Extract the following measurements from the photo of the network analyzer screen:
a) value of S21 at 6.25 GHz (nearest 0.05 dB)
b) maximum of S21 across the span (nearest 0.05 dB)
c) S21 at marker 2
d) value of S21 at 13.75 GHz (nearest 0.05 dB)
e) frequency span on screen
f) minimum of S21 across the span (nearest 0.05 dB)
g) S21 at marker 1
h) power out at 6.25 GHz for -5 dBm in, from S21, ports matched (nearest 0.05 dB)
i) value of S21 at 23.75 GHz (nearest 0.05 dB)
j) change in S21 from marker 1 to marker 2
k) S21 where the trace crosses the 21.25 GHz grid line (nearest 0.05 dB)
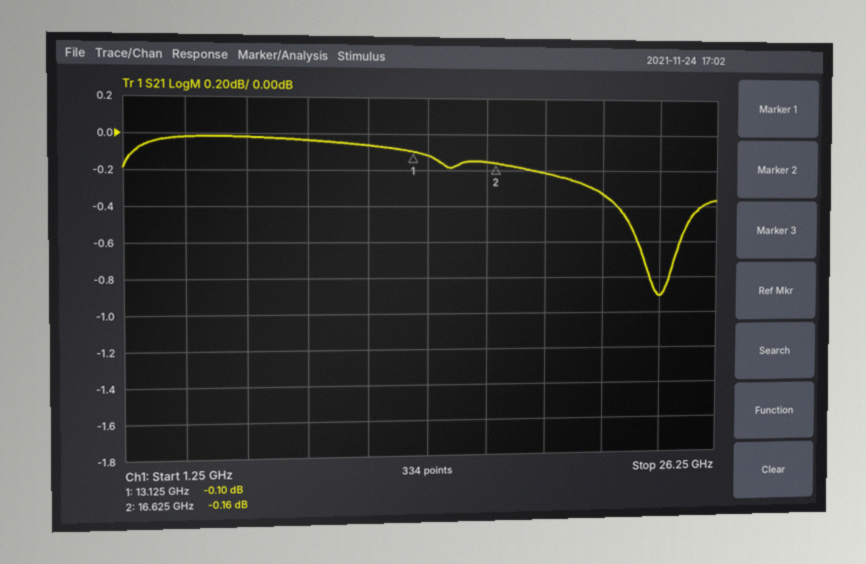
0.00 dB
0.00 dB
-0.16 dB
-0.10 dB
25 GHz
-0.90 dB
-0.10 dB
-5.00 dBm
-0.90 dB
-0.06 dB
-0.35 dB
